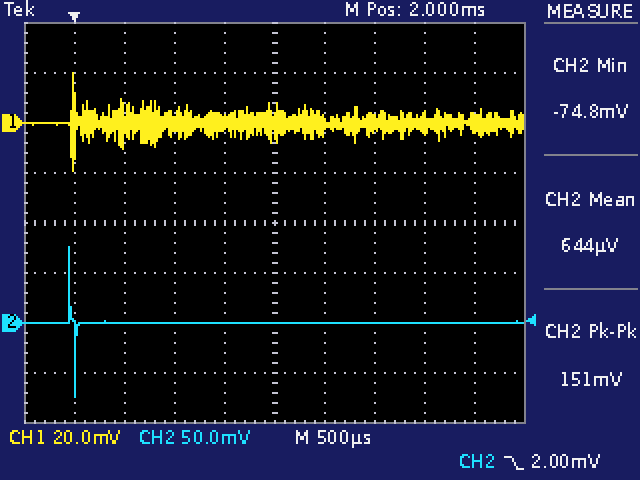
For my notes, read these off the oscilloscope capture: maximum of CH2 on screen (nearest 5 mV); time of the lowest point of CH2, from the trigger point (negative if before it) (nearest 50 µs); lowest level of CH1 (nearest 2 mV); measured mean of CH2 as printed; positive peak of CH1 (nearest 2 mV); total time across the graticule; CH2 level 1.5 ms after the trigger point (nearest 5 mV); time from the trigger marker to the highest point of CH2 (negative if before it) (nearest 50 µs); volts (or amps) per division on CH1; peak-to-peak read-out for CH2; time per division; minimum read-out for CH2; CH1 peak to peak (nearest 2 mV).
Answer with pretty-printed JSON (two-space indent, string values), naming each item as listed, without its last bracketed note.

{
  "maximum of CH2 on screen": "75 mV",
  "time of the lowest point of CH2, from the trigger point (negative if before it)": "0 µs",
  "lowest level of CH1": "-20 mV",
  "measured mean of CH2 as printed": "644 µV",
  "positive peak of CH1": "20 mV",
  "total time across the graticule": "5 ms",
  "CH2 level 1.5 ms after the trigger point": "0 mV",
  "time from the trigger marker to the highest point of CH2 (negative if before it)": "-50 µs",
  "volts (or amps) per division on CH1": "20 mV",
  "peak-to-peak read-out for CH2": "151 mV",
  "time per division": "500 µs",
  "minimum read-out for CH2": "-74.8 mV",
  "CH1 peak to peak": "40 mV"
}
